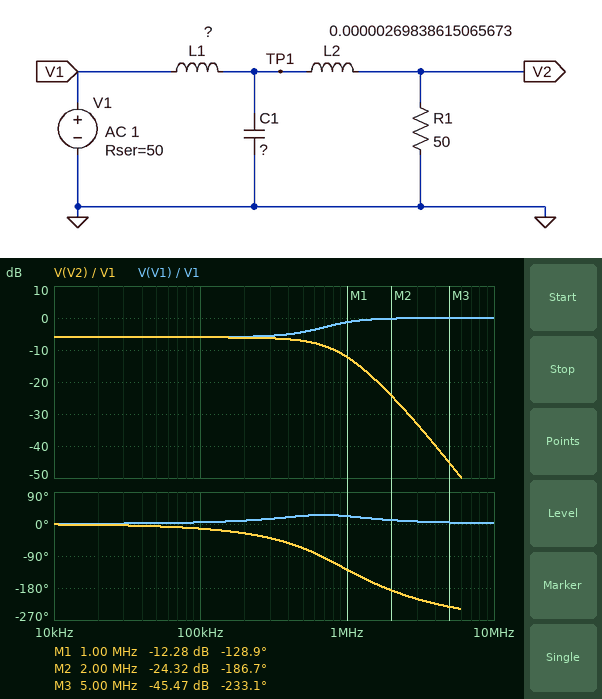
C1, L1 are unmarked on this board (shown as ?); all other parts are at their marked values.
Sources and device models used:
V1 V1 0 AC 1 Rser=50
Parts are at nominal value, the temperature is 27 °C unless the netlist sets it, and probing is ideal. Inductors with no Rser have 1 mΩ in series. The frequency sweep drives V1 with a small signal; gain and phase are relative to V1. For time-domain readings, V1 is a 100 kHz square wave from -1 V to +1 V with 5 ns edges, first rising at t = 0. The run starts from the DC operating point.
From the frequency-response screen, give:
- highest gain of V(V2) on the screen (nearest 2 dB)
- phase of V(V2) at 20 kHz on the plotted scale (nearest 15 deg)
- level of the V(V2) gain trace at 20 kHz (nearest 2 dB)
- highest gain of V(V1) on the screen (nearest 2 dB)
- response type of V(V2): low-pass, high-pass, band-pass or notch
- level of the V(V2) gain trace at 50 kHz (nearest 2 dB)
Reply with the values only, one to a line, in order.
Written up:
-6 dB
0 deg
-6 dB
0 dB
low-pass
-6 dB
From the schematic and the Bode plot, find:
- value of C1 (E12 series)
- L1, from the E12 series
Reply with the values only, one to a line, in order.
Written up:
4.7 nF
22 µH
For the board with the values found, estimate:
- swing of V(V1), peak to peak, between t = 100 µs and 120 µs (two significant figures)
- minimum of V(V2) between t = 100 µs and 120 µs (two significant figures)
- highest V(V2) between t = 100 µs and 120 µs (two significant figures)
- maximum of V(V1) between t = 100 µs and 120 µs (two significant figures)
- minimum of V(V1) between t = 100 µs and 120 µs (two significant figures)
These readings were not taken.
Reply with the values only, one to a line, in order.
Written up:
3.0 V
-520 mV
520 mV
1.5 V
-1.5 V
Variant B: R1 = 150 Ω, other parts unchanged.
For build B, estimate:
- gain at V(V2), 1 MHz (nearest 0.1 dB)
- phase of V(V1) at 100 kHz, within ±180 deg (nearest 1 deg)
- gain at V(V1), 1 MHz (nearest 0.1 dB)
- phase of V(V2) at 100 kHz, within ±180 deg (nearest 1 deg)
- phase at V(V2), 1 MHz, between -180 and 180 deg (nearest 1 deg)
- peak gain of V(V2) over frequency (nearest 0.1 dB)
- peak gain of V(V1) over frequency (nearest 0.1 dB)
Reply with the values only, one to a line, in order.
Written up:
-11.0 dB
-5 deg
-1.1 dB
-11 deg
-145 deg
-1.4 dB
0 dB
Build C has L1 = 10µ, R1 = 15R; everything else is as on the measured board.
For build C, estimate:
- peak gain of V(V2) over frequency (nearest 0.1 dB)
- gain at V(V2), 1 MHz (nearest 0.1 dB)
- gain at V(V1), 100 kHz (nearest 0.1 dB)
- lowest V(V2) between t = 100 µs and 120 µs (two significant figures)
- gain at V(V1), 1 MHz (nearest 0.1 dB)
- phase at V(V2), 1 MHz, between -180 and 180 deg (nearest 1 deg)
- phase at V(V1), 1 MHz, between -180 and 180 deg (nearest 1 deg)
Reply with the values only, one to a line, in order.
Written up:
-12.7 dB
-13.6 dB
-11.8 dB
-260 mV
-3.1 dB
-80 deg
25 deg
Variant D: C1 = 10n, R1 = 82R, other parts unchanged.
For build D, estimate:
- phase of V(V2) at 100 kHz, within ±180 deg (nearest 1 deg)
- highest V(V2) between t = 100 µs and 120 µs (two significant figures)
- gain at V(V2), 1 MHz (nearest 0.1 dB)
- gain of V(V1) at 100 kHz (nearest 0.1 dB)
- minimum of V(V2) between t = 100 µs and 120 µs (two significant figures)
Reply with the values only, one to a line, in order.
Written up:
-18 deg
710 mV
-18.5 dB
-4.7 dB
-710 mV
